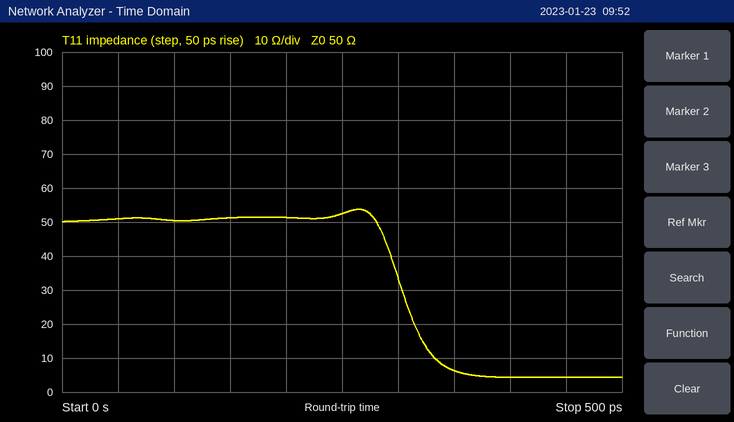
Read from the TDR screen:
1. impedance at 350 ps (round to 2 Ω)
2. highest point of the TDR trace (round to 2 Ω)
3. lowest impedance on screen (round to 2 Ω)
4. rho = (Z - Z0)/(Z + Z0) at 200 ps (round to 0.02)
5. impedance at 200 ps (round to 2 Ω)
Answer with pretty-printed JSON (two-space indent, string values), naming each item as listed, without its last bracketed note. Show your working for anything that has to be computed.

{
  "impedance at 350 ps": "6 Ω",
  "highest point of the TDR trace": "54 Ω",
  "lowest impedance on screen": "4 Ω",
  "rho = (Z - Z0)/(Z + Z0) at 200 ps": "(52 − 50)/(52 + 50) ≈ +0.02",
  "impedance at 200 ps": "52 Ω"
}
